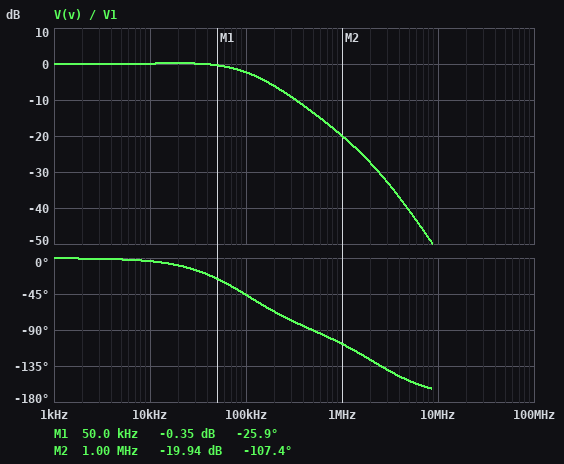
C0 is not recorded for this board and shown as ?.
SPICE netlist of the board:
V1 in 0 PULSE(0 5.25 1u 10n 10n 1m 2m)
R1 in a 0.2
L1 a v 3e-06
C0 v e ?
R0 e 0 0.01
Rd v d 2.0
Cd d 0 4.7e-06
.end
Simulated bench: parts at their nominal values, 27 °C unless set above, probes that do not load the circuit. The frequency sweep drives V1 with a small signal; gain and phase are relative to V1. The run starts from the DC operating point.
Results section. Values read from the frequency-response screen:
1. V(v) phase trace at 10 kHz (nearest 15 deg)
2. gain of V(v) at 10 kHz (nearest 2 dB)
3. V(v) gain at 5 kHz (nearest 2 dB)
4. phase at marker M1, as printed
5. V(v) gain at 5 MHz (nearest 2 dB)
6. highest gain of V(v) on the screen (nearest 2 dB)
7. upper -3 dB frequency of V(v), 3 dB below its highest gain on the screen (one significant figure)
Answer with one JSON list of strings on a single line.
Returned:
["0 deg", "0 dB", "0 dB", "-25.9 deg", "-40 dB", "0 dB", "100 kHz"]
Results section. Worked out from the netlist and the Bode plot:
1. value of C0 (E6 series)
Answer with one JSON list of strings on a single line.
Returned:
["33 nF"]
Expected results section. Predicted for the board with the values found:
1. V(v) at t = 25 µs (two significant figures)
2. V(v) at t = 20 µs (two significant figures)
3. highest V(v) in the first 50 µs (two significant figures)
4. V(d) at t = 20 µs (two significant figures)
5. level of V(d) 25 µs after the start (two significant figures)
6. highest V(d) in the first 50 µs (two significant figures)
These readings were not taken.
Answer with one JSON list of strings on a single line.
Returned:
["5.3 V", "5.3 V", "5.4 V", "4.5 V", "4.8 V", "5.2 V"]
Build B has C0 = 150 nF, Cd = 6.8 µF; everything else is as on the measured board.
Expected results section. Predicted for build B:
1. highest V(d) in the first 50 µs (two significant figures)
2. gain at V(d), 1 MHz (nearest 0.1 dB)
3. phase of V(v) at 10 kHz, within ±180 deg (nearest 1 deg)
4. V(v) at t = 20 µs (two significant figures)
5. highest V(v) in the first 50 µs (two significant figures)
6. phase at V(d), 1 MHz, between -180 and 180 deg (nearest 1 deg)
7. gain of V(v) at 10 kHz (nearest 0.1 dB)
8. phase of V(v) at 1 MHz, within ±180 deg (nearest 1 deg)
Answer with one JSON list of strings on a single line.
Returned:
["5.1 V", "-64.4 dB", "-5 deg", "5.3 V", "5.3 V", "121 deg", "0 dB", "-150 deg"]
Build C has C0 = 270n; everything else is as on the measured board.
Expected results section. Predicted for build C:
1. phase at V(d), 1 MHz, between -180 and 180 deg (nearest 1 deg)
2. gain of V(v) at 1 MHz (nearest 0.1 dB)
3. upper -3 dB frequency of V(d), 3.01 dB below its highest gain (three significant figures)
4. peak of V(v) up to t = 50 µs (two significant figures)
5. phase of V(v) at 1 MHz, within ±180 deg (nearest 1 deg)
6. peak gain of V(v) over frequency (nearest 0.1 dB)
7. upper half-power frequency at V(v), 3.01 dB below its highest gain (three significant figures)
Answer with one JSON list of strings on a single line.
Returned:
["109 deg", "-30.3 dB", "18.0 kHz", "5.5 V", "-162 deg", "0.3 dB", "135 kHz"]
